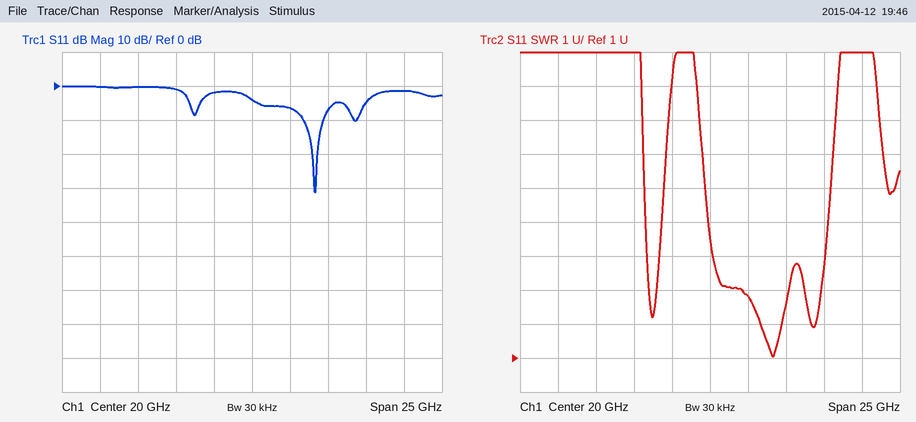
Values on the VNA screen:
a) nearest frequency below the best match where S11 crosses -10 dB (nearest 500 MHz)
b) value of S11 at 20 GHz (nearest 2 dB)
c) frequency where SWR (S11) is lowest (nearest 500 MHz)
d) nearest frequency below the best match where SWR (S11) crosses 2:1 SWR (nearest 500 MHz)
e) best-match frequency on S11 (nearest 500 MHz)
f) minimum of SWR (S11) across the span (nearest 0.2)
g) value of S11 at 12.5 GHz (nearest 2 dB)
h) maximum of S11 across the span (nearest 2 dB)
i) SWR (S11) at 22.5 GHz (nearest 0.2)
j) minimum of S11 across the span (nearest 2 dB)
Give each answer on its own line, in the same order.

23.5 GHz
-4 dB
24.0 GHz
23.5 GHz
24.0 GHz
1.0
0 dB
0 dB
2.8
-32 dB
